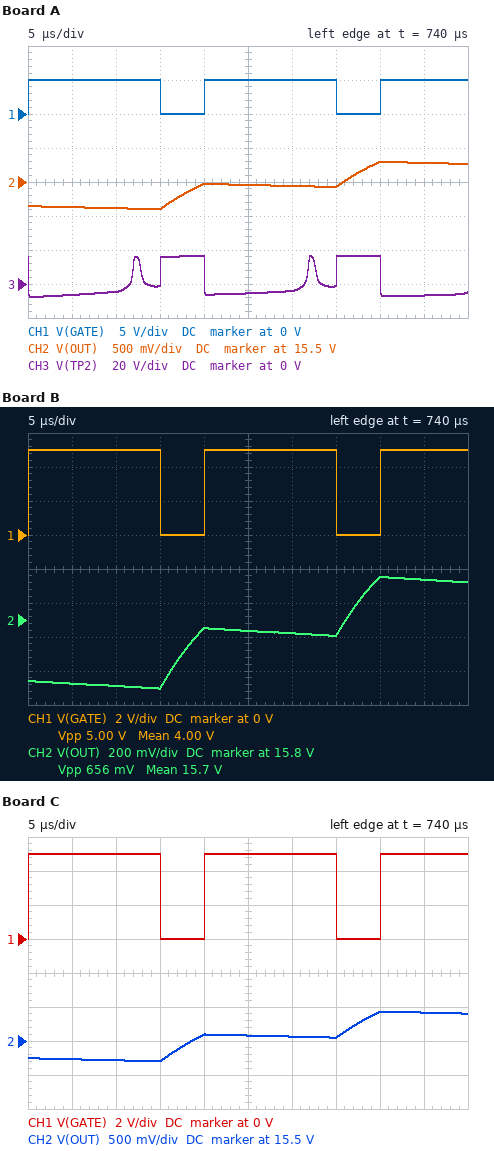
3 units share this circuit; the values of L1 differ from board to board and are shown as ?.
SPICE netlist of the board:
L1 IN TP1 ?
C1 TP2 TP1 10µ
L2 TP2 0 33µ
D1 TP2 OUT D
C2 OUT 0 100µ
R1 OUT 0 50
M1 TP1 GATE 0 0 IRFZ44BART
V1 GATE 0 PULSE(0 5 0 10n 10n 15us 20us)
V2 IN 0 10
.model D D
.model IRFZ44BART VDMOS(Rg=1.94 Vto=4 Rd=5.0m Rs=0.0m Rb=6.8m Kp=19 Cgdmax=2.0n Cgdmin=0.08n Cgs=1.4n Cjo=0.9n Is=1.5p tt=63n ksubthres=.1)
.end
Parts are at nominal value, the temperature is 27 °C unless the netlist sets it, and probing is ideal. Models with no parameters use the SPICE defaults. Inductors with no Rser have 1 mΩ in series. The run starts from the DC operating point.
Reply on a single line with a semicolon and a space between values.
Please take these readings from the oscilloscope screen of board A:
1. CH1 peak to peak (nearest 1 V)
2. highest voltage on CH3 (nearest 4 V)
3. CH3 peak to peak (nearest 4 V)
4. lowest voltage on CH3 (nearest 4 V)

5 V; 16 V; 24 V; -8 V
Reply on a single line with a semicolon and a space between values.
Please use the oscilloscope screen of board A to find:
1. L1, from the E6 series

47 µH
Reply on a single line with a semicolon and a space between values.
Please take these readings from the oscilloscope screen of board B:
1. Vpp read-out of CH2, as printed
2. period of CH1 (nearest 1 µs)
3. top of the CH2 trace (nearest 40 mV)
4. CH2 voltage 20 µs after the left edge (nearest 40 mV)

656 mV; 20 µs; 16.04 V; 15.76 V
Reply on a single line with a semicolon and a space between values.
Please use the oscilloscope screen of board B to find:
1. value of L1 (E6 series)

68 µH
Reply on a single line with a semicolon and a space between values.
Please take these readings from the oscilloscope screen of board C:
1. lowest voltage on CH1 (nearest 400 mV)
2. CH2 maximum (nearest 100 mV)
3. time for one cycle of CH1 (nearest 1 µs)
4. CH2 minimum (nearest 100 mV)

0 V; 15.9 V; 20 µs; 15.2 V
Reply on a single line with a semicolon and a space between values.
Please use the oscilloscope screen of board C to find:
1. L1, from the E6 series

100 µH
